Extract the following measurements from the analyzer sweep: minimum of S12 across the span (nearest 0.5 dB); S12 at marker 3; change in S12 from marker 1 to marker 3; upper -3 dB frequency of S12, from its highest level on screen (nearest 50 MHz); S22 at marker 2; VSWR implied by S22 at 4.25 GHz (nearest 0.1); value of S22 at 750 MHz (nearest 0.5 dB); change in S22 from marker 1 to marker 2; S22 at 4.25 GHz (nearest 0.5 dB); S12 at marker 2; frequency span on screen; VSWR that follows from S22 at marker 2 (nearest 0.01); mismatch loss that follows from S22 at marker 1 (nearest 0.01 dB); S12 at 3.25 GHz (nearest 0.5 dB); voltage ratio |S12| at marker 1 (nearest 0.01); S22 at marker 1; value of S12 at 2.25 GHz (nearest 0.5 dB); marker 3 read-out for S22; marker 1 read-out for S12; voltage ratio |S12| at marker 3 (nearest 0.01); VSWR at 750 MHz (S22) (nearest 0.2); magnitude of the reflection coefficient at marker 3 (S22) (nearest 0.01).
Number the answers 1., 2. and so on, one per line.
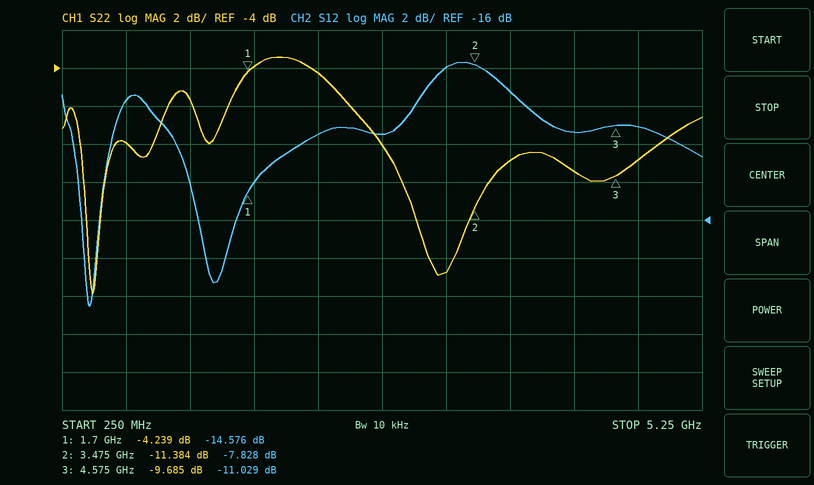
1. -20.5 dB
2. -11.029 dB
3. 3.547 dB
4. 4.00 GHz
5. -11.384 dB
6. 2.0
7. -8.0 dB
8. -7.145 dB
9. -9.5 dB
10. -7.828 dB
11. 5 GHz
12. 1.74
13. 2.05 dB
14. -8.0 dB
15. 0.19
16. -4.239 dB
17. -11.5 dB
18. -9.685 dB
19. -14.576 dB
20. 0.28
21. 2.4
22. 0.33
